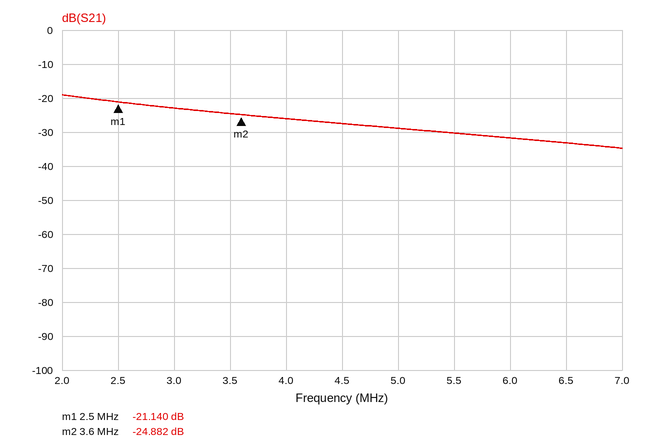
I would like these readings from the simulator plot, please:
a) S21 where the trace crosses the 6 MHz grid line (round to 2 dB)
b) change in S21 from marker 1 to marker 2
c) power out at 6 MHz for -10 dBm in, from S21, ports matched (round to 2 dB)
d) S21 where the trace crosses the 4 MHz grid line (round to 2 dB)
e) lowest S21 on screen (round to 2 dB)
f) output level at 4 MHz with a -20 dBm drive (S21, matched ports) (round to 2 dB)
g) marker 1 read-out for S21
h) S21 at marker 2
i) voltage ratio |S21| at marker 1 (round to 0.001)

-32 dB
-3.742 dB
-42 dBm
-26 dB
-34 dB
-46 dBm
-21.140 dB
-24.882 dB
0.088
